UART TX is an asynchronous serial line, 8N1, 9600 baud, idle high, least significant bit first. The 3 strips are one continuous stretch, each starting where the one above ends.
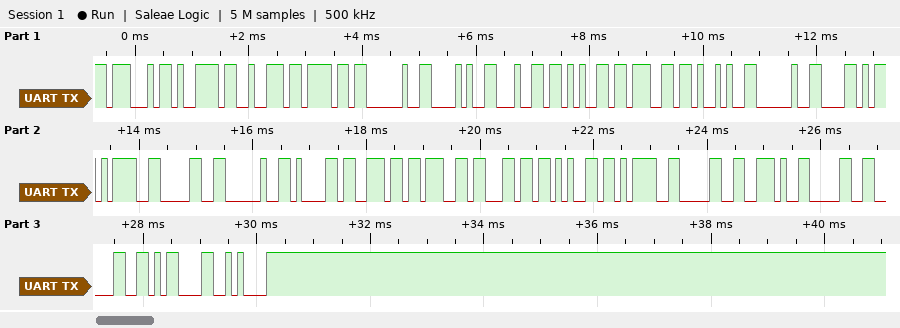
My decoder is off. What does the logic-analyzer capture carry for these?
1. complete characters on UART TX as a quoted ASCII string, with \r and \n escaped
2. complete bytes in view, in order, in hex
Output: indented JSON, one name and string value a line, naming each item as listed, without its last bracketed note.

{
  "complete characters on UART TX as a quoted ASCII string, with \\r and \\n escaped": "\"Gyro (deg) X=0 angle=0.00\\r\\n\"",
  "complete bytes in view, in order, in hex": "47 79 72 6F 20 28 64 65 67 29 20 58 3D 30 20 61 6E 67 6C 65 3D 30 2E 30 30 0D 0A"
}
